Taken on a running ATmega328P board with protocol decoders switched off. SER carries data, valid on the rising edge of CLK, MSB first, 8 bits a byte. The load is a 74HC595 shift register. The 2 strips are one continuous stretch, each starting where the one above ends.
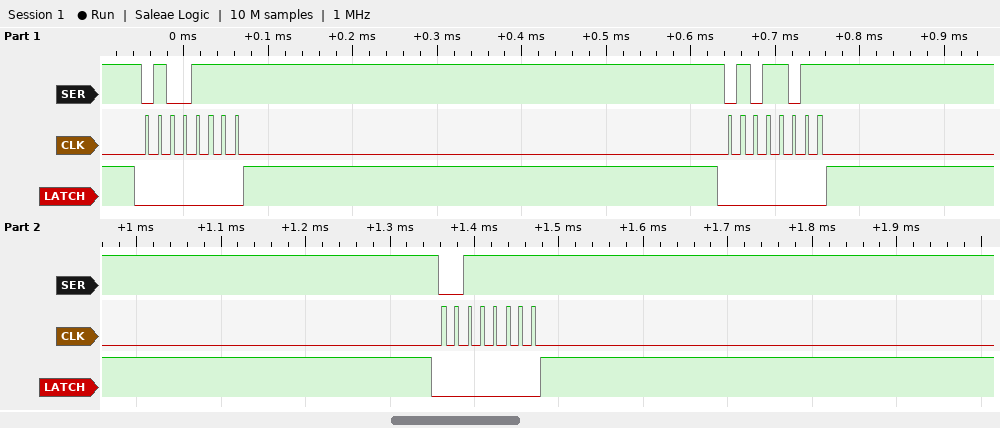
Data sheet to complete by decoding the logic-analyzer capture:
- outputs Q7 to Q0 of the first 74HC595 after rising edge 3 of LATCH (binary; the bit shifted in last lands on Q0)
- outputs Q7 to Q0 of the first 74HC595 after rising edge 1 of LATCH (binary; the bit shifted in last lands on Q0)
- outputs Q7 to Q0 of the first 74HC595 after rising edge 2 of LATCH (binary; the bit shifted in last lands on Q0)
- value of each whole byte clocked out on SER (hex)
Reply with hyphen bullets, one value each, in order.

- 00111111
- 01001111
- 01011011
- 4F 5B 3F
